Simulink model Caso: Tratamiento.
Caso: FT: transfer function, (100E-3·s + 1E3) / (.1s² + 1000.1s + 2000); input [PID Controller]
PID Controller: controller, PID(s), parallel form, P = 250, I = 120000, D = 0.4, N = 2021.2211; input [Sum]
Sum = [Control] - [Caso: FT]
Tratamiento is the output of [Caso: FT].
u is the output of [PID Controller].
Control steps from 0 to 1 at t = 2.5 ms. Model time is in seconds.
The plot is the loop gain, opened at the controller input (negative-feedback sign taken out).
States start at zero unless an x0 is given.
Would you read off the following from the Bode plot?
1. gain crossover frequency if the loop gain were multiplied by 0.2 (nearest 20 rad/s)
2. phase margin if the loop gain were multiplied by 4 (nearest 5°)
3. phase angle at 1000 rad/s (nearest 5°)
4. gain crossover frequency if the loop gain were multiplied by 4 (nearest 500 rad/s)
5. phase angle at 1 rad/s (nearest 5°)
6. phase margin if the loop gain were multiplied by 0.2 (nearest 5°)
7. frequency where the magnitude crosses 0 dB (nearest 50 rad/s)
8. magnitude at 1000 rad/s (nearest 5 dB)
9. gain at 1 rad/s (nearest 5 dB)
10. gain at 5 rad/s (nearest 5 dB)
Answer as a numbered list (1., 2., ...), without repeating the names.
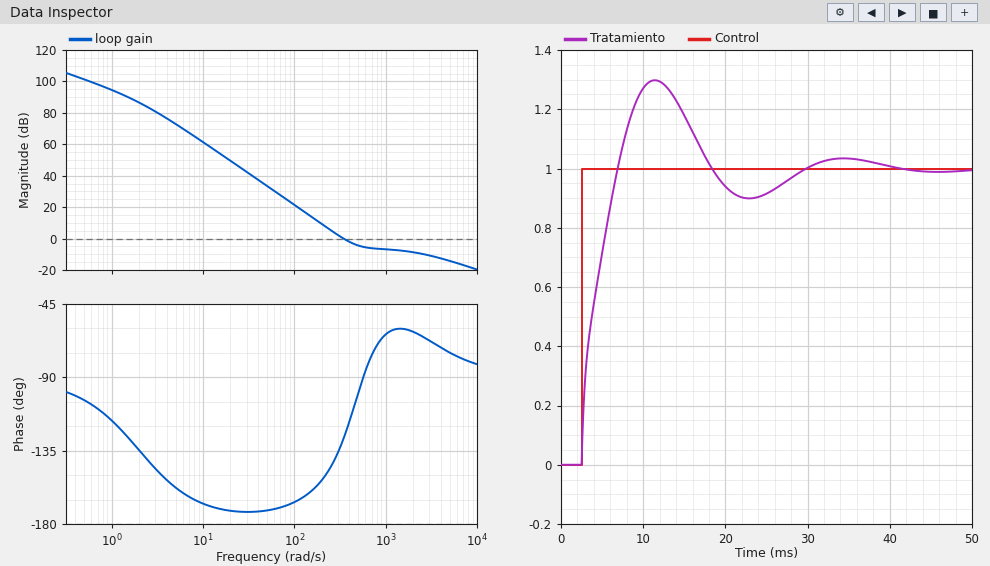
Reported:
1. 160 rad/s
2. 110°
3. -65°
4. 3500 rad/s
5. -115°
6. 20°
7. 350 rad/s
8. -5 dB
9. 95 dB
10. 75 dB
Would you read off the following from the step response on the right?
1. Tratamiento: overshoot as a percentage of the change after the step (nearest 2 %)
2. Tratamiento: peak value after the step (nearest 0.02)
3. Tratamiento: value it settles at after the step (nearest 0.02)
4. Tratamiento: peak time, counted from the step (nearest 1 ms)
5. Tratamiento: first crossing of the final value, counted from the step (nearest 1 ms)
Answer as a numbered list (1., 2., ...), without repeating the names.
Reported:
1. 30 %
2. 1.30
3. 1.00
4. 9 ms
5. 4 ms
